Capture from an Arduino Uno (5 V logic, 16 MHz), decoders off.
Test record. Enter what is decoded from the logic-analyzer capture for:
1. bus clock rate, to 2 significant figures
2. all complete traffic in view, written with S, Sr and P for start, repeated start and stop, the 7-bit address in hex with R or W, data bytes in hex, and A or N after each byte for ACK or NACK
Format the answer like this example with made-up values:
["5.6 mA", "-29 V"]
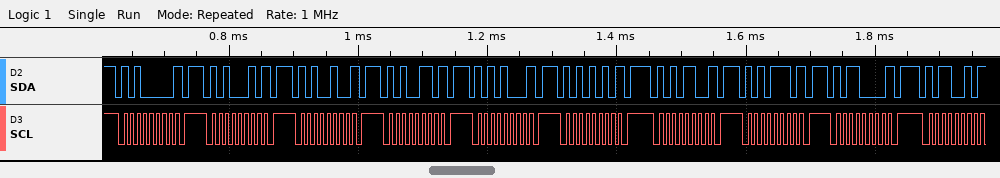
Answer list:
["100 kHz", "S 50W N P S 51W N P S 52W N P S 53W N P S 54W N P S 55W N P S 56W N P S 57W N P S 58W N P S 59W N"]
